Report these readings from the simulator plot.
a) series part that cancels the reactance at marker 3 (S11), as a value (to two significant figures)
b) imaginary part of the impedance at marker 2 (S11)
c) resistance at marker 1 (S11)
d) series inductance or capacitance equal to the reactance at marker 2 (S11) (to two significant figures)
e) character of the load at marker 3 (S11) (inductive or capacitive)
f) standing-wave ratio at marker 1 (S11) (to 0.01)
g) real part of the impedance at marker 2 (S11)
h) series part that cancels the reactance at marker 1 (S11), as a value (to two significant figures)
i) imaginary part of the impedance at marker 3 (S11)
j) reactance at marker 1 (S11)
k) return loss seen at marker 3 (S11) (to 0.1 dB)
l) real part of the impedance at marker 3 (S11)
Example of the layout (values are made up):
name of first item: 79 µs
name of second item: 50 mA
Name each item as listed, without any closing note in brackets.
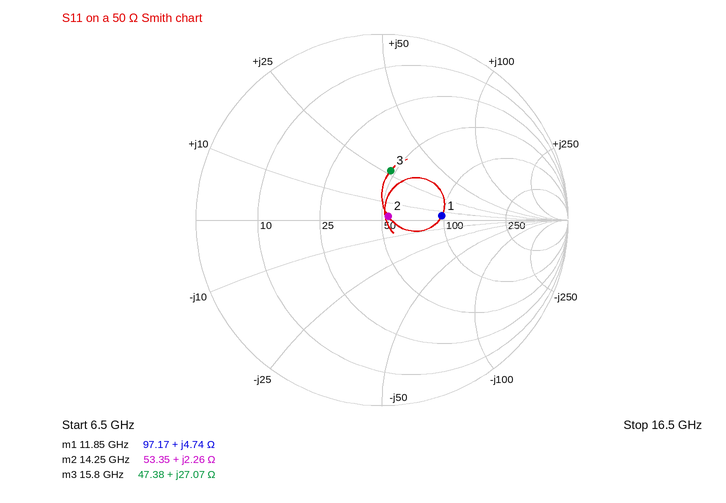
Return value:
series part that cancels the reactance at marker 3 (S11), as a value: 370 fF
imaginary part of the impedance at marker 2: +2.26 Ω
resistance at marker 1: 97.17 Ω
series inductance or capacitance equal to the reactance at marker 2 (S11): 25 pH
character of the load at marker 3 (S11): inductive
standing-wave ratio at marker 1 (S11): 1.95
real part of the impedance at marker 2: 53.35 Ω
series part that cancels the reactance at marker 1 (S11), as a value: 2.8 pF
imaginary part of the impedance at marker 3: +27.07 Ω
reactance at marker 1: +4.74 Ω
return loss seen at marker 3 (S11): 11.4 dB
real part of the impedance at marker 3: 47.38 Ω
